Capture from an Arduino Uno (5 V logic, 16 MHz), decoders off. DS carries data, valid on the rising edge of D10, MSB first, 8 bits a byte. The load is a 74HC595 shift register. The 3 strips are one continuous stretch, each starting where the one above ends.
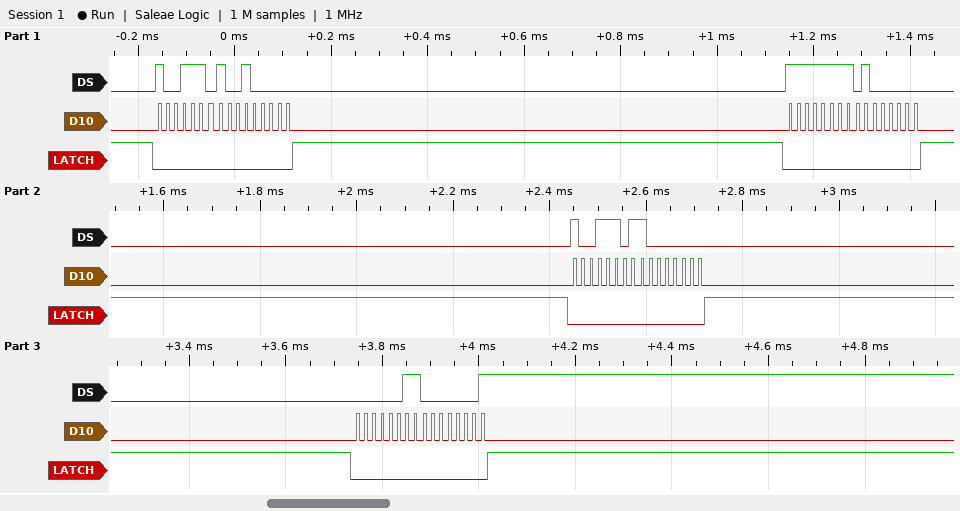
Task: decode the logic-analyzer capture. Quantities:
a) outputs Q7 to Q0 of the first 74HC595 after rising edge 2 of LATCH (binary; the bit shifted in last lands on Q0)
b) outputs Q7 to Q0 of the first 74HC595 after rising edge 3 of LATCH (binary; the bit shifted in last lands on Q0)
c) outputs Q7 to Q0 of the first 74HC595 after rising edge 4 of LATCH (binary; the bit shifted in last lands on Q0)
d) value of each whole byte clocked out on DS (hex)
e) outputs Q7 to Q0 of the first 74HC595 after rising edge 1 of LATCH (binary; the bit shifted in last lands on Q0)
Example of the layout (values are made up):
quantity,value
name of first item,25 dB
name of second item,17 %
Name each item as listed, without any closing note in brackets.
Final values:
quantity,value
outputs Q7 to Q0 of the first 74HC595 after rising edge 2 of LATCH,01000000
outputs Q7 to Q0 of the first 74HC595 after rising edge 3 of LATCH,10000000
outputs Q7 to Q0 of the first 74HC595 after rising edge 4 of LATCH,00000001
value of each whole byte clocked out on DS,9D 20 FF 40 9D 80 03 01
outputs Q7 to Q0 of the first 74HC595 after rising edge 1 of LATCH,00100000
